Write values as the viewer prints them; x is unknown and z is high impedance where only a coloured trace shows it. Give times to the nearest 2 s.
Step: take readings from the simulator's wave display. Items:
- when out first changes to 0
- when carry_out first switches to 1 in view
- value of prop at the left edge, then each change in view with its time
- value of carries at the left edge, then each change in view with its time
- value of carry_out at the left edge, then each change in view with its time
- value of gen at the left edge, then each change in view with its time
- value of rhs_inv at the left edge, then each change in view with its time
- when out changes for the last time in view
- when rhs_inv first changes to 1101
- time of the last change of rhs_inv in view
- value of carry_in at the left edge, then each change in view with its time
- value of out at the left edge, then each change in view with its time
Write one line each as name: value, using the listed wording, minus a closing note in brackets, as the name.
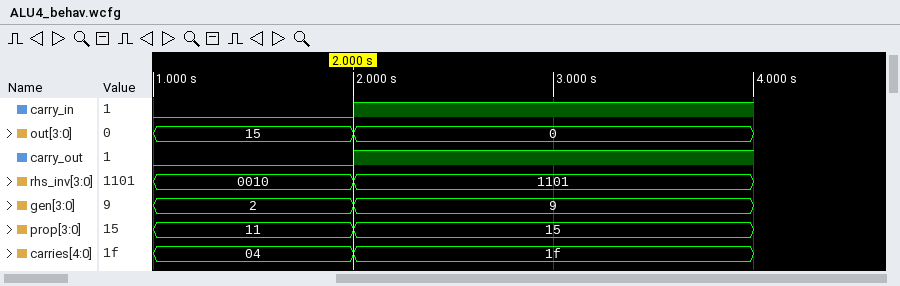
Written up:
when out first changes to 0: 2 s
when carry_out first switches to 1 in view: 2 s
value of prop at the left edge, then each change in view with its time: 11, 15 at 2 s
value of carries at the left edge, then each change in view with its time: 04, 1f at 2 s
value of carry_out at the left edge, then each change in view with its time: 0, 1 at 2 s
value of gen at the left edge, then each change in view with its time: 2, 9 at 2 s
value of rhs_inv at the left edge, then each change in view with its time: 0010, 1101 at 2 s
when out changes for the last time in view: 2 s
when rhs_inv first changes to 1101: 2 s
time of the last change of rhs_inv in view: 2 s
value of carry_in at the left edge, then each change in view with its time: 0, 1 at 2 s
value of out at the left edge, then each change in view with its time: 15, 0 at 2 s
